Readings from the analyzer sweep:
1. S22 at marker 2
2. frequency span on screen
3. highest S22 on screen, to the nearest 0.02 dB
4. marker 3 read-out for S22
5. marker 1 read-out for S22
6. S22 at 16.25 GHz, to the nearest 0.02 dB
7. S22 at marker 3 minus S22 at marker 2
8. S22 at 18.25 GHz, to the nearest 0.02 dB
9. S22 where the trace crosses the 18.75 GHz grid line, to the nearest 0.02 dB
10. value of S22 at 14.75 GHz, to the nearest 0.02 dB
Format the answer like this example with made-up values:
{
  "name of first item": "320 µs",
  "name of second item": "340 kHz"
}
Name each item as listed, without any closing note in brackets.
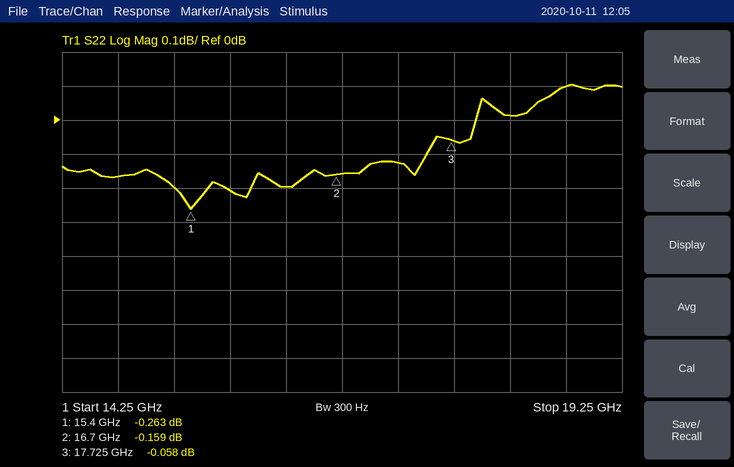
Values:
{
  "S22 at marker 2": "-0.159 dB",
  "frequency span on screen": "5 GHz",
  "highest S22 on screen, to the nearest 0.02 dB": "0.10 dB",
  "marker 3 read-out for S22": "-0.058 dB",
  "marker 1 read-out for S22": "-0.263 dB",
  "S22 at 16.25 GHz, to the nearest 0.02 dB": "-0.20 dB",
  "S22 at marker 3 minus S22 at marker 2": "0.101 dB",
  "S22 at 18.25 GHz, to the nearest 0.02 dB": "0.02 dB",
  "S22 where the trace crosses the 18.75 GHz grid line, to the nearest 0.02 dB": "0.10 dB",
  "value of S22 at 14.75 GHz, to the nearest 0.02 dB": "-0.16 dB"
}
